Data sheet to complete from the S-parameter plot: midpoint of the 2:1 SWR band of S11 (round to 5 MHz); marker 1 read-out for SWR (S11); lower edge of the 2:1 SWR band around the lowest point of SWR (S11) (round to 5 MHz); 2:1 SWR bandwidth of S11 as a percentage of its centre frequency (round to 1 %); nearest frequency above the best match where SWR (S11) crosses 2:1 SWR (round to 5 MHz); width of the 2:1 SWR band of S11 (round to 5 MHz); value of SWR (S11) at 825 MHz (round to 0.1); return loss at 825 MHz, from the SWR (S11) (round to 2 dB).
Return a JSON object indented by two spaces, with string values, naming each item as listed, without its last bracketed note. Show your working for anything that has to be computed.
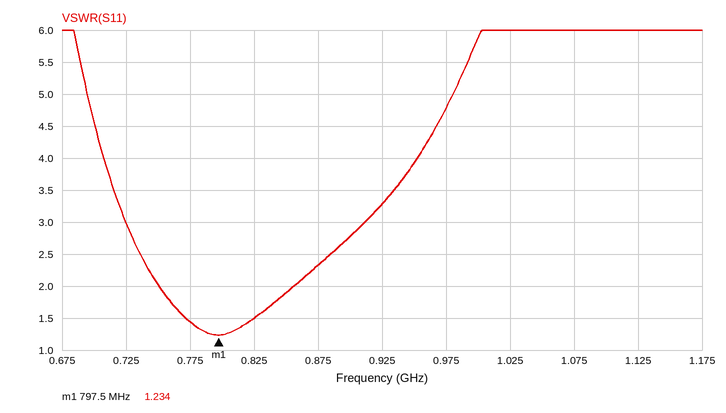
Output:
{
  "midpoint of the 2:1 SWR band of S11": "805 MHz",
  "marker 1 read-out for SWR": "1.234",
  "lower edge of the 2:1 SWR band around the lowest point of SWR (S11)": "750 MHz",
  "2:1 SWR bandwidth of S11 as a percentage of its centre frequency": "105 MHz / 802.5 MHz ≈ 13 %",
  "nearest frequency above the best match where SWR (S11) crosses 2:1 SWR": "855 MHz",
  "width of the 2:1 SWR band of S11": "855 MHz − 750 MHz = 105 MHz",
  "value of SWR (S11) at 825 MHz": "1.5",
  "return loss at 825 MHz, from the SWR (S11)": "−20 log10((1.5 − 1)/(1.5 + 1)) ≈ 14 dB"
}
